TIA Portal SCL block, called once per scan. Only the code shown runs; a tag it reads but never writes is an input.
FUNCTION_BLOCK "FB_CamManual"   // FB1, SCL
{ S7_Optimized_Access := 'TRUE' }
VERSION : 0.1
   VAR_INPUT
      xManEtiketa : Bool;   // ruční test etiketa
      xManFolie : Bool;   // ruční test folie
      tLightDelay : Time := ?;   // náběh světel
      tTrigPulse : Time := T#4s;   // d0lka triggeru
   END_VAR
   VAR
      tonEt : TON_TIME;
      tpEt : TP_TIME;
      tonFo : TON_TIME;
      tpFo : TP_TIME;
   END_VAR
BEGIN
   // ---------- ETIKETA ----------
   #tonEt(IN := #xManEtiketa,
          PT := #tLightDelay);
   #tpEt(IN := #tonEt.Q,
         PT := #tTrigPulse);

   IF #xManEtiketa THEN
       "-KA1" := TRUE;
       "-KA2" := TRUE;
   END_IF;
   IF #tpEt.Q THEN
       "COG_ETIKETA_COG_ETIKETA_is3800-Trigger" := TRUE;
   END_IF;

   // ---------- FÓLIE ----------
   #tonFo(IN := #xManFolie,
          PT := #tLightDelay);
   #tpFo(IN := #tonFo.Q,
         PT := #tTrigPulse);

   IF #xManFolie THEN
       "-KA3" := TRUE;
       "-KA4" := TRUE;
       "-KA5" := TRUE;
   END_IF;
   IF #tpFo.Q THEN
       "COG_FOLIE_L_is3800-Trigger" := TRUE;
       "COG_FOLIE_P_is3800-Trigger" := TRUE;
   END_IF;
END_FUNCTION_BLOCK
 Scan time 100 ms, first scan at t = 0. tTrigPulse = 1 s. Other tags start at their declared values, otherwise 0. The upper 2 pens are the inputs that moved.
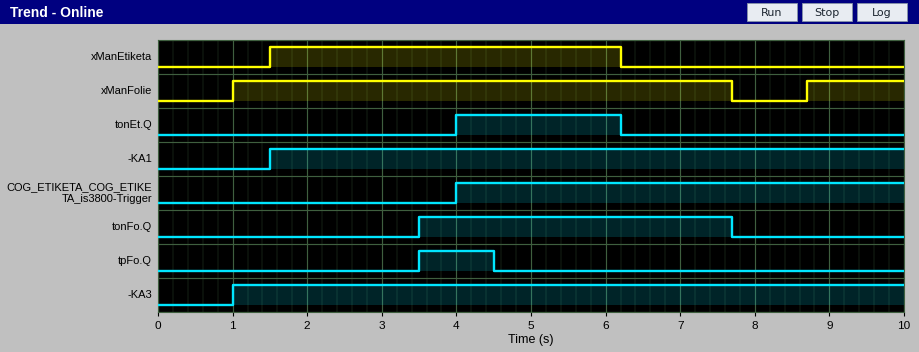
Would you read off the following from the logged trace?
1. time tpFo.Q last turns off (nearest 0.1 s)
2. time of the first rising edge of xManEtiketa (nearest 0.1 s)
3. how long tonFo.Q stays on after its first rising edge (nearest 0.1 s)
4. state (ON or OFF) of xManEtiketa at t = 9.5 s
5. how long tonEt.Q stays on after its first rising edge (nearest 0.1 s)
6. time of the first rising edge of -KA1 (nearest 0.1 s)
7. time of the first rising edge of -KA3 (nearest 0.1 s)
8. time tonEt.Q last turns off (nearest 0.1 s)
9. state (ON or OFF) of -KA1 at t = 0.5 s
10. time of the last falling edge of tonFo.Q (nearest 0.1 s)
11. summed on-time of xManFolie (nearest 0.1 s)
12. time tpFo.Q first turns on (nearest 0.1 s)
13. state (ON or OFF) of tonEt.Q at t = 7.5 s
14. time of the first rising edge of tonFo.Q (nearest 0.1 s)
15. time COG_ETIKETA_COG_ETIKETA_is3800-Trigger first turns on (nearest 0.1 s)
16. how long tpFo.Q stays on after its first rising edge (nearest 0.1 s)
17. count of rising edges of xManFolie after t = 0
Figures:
4.5 s
1.5 s
4.2 s
OFF
2.2 s
1.5 s
1.0 s
6.2 s
OFF
7.7 s
8.0 s
3.5 s
OFF
3.5 s
4.0 s
1.0 s
2
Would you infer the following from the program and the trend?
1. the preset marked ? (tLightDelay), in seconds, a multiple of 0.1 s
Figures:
2.5 s
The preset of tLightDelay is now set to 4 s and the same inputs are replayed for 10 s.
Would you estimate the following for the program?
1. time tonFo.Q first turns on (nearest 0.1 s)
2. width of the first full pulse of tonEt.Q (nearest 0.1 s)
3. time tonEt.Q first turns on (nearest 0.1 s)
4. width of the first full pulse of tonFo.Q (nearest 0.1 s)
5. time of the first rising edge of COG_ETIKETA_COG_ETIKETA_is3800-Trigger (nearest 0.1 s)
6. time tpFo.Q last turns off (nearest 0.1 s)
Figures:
5.0 s
0.7 s
5.5 s
2.7 s
5.5 s
6.0 s
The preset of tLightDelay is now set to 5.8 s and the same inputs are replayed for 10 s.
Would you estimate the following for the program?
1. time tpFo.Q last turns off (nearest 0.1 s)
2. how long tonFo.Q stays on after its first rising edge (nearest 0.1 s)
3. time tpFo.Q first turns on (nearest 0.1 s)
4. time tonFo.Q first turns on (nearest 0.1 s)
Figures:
7.8 s
0.9 s
6.8 s
6.8 s
